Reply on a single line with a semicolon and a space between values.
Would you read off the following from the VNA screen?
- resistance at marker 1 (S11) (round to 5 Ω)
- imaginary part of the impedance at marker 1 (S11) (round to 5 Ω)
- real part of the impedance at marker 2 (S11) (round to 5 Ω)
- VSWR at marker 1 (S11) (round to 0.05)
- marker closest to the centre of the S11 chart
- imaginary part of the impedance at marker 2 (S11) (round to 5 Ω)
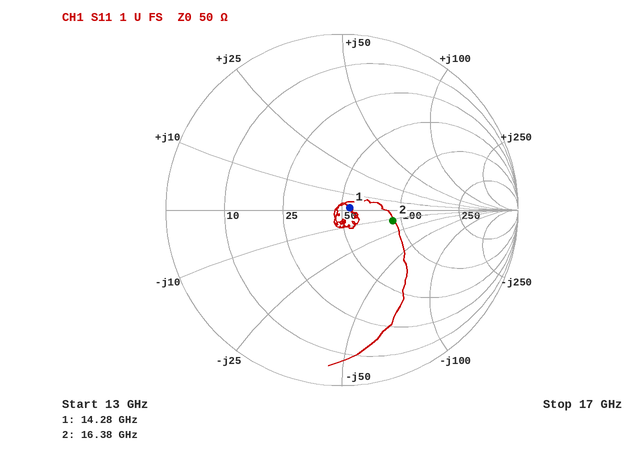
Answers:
55 Ω; 0 Ω; 90 Ω; 1.10; marker 1; -10 Ω
